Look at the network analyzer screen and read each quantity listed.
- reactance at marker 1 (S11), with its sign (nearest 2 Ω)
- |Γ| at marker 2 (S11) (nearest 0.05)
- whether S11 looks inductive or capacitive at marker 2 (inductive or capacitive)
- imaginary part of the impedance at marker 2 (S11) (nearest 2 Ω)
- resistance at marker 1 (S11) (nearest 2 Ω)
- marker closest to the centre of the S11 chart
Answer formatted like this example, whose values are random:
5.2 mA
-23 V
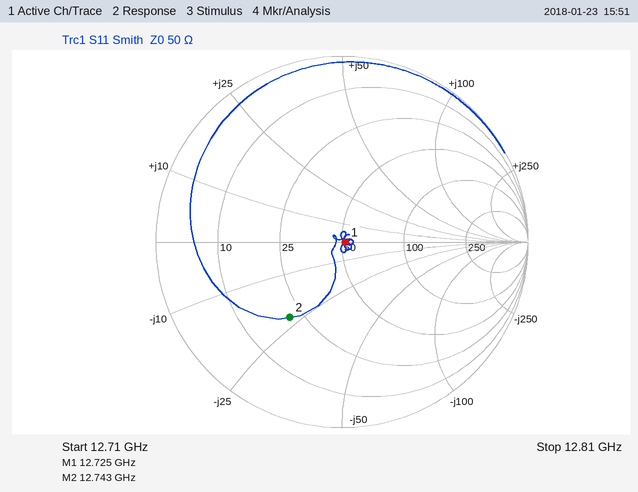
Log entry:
0 Ω
0.50
capacitive
-22 Ω
52 Ω
marker 1
